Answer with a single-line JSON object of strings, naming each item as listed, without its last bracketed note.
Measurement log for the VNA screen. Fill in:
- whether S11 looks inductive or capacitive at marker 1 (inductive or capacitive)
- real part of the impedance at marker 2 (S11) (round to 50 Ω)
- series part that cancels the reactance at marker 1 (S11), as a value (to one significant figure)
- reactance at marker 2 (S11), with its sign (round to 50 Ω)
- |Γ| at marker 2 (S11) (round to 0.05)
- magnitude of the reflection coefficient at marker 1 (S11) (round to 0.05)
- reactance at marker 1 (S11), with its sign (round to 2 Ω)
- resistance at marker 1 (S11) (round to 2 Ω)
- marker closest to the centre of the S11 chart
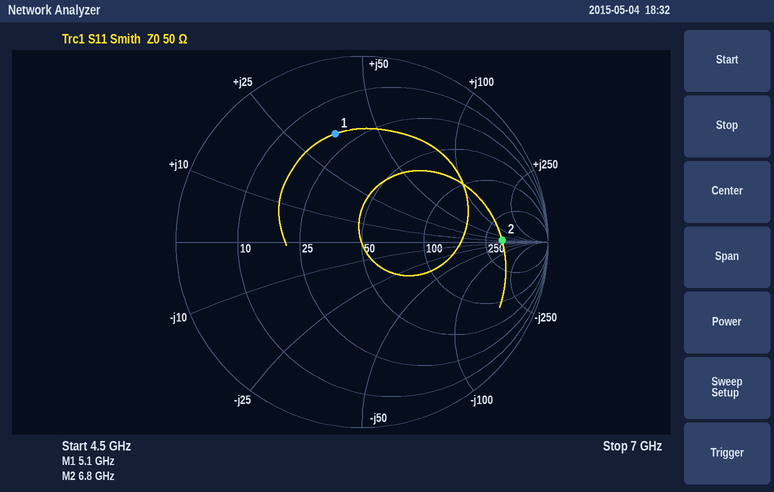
{"whether S11 looks inductive or capacitive at marker 1": "inductive", "real part of the impedance at marker 2 (S11)": "350 Ω", "series part that cancels the reactance at marker 1 (S11), as a value": "900 fF", "reactance at marker 2 (S11), with its sign": "0 Ω", "|Γ| at marker 2 (S11)": "0.75", "magnitude of the reflection coefficient at marker 1 (S11)": "0.60", "reactance at marker 1 (S11), with its sign": "+36 Ω", "resistance at marker 1 (S11)": "20 Ω", "marker closest to the centre of the S11 chart": "marker 1"}
